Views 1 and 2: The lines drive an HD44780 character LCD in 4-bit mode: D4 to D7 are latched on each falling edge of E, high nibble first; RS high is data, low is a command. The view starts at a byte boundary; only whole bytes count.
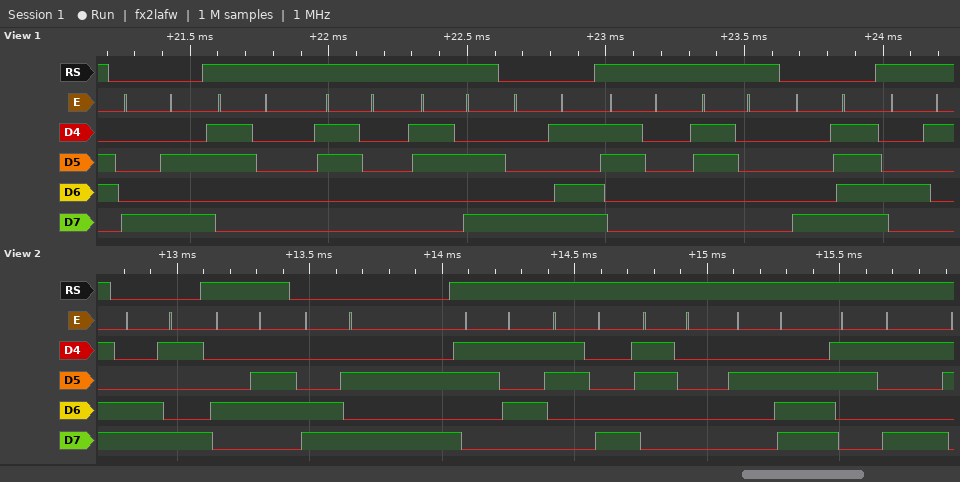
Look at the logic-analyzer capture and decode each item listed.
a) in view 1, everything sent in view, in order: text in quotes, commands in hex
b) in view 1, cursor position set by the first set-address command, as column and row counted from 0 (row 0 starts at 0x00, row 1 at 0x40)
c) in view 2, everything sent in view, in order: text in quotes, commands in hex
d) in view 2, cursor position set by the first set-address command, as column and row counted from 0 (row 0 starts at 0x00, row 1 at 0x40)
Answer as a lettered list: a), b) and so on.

a) 0x8A "00:" 0x8D "00" 0x8F "A"
b) column 10, row 0
c) 0xC9 "F" 0xCA "580.9"
d) column 9, row 1
